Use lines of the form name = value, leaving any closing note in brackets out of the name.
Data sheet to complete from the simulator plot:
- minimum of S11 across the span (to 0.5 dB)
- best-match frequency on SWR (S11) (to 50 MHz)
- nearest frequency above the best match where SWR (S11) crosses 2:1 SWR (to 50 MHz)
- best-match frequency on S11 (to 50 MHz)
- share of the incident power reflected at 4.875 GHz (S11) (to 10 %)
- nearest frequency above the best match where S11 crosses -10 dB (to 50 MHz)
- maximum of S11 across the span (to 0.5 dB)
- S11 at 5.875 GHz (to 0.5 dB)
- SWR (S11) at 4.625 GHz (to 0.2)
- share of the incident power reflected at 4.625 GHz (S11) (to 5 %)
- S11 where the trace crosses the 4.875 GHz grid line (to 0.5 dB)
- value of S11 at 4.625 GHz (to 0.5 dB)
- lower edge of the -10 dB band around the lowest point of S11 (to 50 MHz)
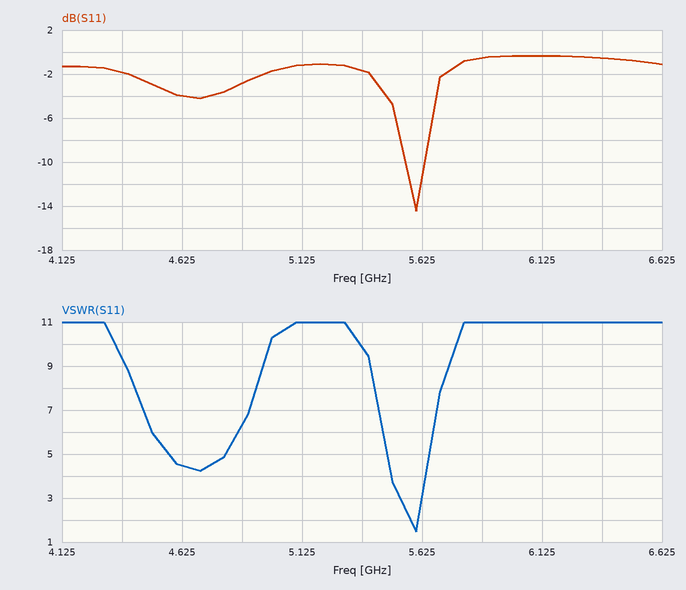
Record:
minimum of S11 across the span = -14.5 dB
best-match frequency on SWR (S11) = 5.60 GHz
nearest frequency above the best match where SWR (S11) crosses 2:1 SWR = 5.60 GHz
best-match frequency on S11 = 5.60 GHz
share of the incident power reflected at 4.875 GHz (S11) = 50 %
nearest frequency above the best match where S11 crosses -10 dB = 5.65 GHz
maximum of S11 across the span = -0.5 dB
S11 at 5.875 GHz = -0.5 dB
SWR (S11) at 4.625 GHz = 4.4
share of the incident power reflected at 4.625 GHz (S11) = 40 %
S11 where the trace crosses the 4.875 GHz grid line = -3.0 dB
value of S11 at 4.625 GHz = -4.0 dB
lower edge of the -10 dB band around the lowest point of S11 = 5.55 GHz
